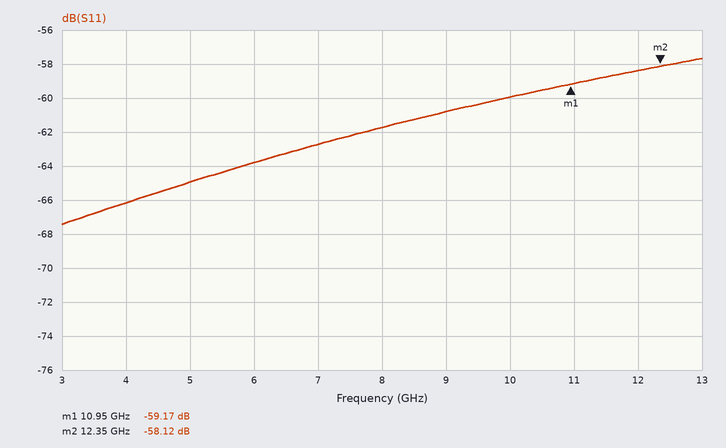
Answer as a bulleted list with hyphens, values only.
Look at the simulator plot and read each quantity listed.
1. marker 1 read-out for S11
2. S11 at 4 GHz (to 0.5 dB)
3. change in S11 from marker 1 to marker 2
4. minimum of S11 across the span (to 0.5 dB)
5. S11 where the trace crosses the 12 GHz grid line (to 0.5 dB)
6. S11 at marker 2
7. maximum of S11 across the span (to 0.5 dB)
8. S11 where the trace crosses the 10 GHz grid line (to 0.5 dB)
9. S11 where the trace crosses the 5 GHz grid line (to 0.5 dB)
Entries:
- -59.17 dB
- -66.0 dB
- 1.05 dB
- -67.5 dB
- -58.5 dB
- -58.12 dB
- -57.5 dB
- -60.0 dB
- -65.0 dB
